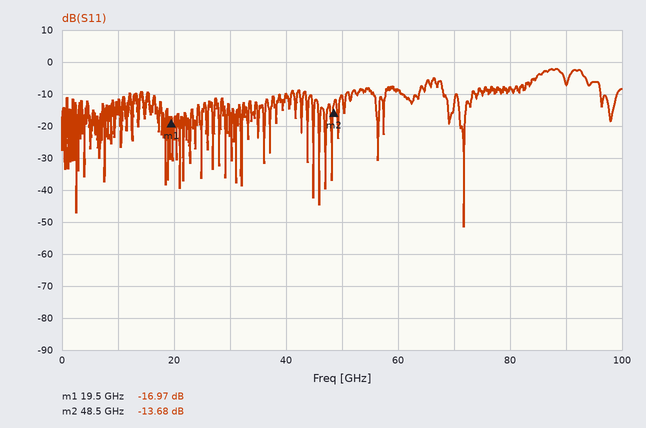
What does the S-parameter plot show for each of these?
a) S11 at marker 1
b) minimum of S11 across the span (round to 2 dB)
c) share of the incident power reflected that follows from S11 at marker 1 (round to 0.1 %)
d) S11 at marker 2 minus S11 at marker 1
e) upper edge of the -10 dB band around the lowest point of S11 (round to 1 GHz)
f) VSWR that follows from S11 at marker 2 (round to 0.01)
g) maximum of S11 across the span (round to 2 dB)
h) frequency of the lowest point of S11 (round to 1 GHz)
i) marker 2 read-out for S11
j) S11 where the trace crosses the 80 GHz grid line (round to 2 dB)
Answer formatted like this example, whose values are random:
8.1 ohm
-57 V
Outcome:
-16.97 dB
-52 dB
2.0 %
3.29 dB
73 GHz
1.52
-2 dB
72 GHz
-13.68 dB
-8 dB
